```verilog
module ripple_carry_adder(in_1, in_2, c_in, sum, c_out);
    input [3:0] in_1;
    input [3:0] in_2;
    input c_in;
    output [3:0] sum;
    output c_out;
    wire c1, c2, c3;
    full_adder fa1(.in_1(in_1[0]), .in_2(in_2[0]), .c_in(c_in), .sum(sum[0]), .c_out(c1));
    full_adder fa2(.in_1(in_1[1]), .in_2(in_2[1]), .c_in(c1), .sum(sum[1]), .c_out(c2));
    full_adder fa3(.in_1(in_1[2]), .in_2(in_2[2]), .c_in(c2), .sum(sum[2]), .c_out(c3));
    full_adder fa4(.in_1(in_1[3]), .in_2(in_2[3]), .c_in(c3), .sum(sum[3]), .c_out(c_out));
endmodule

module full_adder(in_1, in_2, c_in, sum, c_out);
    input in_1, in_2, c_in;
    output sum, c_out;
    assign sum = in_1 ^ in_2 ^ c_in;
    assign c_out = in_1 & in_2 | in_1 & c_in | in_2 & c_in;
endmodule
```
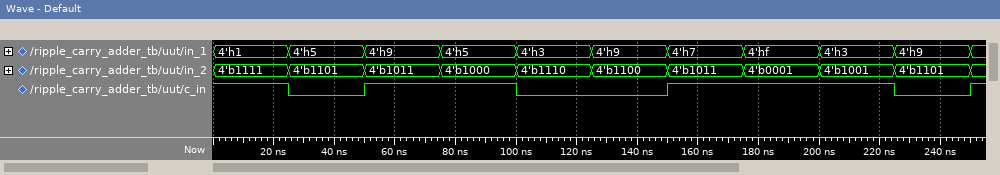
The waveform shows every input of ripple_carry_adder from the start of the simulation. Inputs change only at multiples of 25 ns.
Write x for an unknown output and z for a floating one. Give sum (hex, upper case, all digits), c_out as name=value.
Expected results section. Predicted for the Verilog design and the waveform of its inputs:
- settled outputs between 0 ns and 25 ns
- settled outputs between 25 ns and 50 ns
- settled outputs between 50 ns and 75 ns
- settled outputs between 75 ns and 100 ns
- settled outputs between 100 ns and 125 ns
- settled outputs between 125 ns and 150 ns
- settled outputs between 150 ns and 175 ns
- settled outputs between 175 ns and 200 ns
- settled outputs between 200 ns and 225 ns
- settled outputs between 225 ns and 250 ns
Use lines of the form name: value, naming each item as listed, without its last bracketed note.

settled outputs between 0 ns and 25 ns: sum=1, c_out=1
settled outputs between 25 ns and 50 ns: sum=2, c_out=1
settled outputs between 50 ns and 75 ns: sum=5, c_out=1
settled outputs between 75 ns and 100 ns: sum=E, c_out=0
settled outputs between 100 ns and 125 ns: sum=1, c_out=1
settled outputs between 125 ns and 150 ns: sum=5, c_out=1
settled outputs between 150 ns and 175 ns: sum=3, c_out=1
settled outputs between 175 ns and 200 ns: sum=1, c_out=1
settled outputs between 200 ns and 225 ns: sum=D, c_out=0
settled outputs between 225 ns and 250 ns: sum=6, c_out=1
